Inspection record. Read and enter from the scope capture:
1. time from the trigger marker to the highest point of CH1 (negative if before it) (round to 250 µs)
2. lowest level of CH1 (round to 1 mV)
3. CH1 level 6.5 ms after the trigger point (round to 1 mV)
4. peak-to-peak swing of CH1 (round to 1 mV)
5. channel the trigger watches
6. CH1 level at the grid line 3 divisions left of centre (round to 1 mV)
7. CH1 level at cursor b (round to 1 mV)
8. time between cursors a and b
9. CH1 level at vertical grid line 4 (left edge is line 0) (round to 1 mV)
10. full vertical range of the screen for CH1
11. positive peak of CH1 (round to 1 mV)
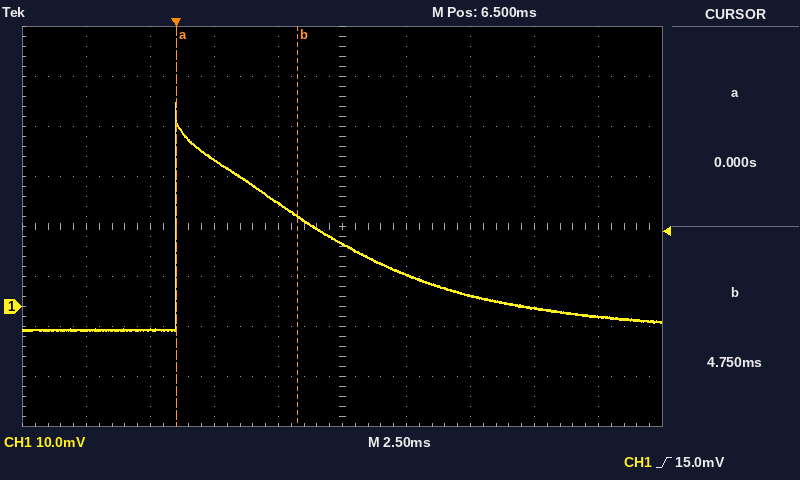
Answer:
0.00 ms
-5 mV
13 mV
46 mV
CH1
-5 mV
18 mV
4.75 ms
21 mV
80 mV
41 mV
